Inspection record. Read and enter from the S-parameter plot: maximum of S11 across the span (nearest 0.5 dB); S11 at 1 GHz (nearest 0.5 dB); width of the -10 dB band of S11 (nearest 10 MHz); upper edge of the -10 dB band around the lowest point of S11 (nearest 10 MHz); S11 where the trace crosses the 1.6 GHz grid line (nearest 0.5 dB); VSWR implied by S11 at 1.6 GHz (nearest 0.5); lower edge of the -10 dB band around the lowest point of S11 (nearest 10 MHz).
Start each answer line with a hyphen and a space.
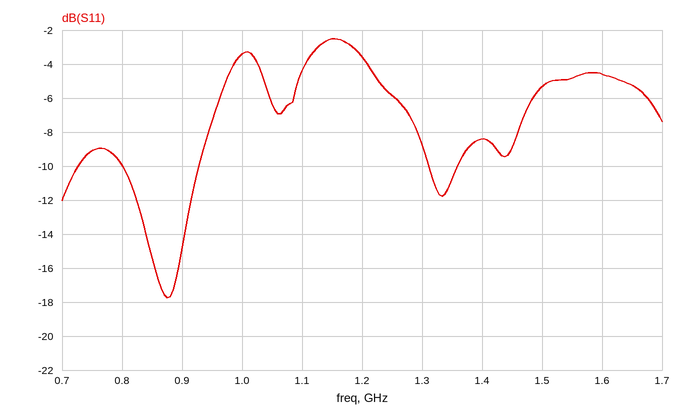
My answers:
- -2.5 dB
- -3.5 dB
- 130 MHz
- 930 MHz
- -4.5 dB
- 4.0
- 800 MHz
